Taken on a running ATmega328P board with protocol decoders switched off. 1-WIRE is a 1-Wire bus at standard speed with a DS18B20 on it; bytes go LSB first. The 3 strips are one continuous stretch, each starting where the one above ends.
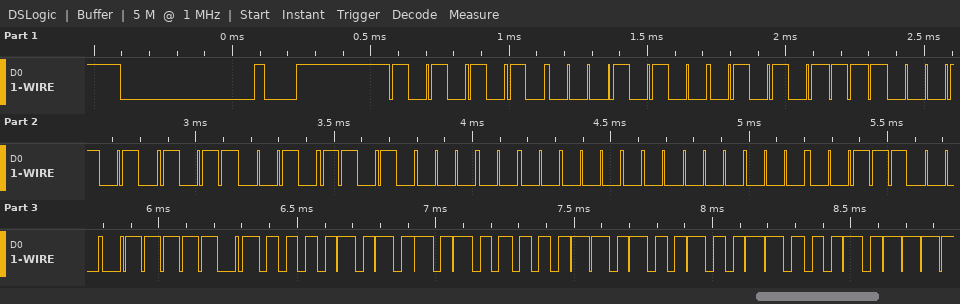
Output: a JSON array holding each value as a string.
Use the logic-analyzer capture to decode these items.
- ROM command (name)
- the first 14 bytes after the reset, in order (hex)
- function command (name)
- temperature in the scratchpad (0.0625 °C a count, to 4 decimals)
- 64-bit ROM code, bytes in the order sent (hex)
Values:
["Match ROM", "55 28 EA 51 4D 0B 00 00 1C BE 50 05 4B 46", "Read Scratchpad", "85.0000 °C", "28 EA 51 4D 0B 00 00 1C"]
